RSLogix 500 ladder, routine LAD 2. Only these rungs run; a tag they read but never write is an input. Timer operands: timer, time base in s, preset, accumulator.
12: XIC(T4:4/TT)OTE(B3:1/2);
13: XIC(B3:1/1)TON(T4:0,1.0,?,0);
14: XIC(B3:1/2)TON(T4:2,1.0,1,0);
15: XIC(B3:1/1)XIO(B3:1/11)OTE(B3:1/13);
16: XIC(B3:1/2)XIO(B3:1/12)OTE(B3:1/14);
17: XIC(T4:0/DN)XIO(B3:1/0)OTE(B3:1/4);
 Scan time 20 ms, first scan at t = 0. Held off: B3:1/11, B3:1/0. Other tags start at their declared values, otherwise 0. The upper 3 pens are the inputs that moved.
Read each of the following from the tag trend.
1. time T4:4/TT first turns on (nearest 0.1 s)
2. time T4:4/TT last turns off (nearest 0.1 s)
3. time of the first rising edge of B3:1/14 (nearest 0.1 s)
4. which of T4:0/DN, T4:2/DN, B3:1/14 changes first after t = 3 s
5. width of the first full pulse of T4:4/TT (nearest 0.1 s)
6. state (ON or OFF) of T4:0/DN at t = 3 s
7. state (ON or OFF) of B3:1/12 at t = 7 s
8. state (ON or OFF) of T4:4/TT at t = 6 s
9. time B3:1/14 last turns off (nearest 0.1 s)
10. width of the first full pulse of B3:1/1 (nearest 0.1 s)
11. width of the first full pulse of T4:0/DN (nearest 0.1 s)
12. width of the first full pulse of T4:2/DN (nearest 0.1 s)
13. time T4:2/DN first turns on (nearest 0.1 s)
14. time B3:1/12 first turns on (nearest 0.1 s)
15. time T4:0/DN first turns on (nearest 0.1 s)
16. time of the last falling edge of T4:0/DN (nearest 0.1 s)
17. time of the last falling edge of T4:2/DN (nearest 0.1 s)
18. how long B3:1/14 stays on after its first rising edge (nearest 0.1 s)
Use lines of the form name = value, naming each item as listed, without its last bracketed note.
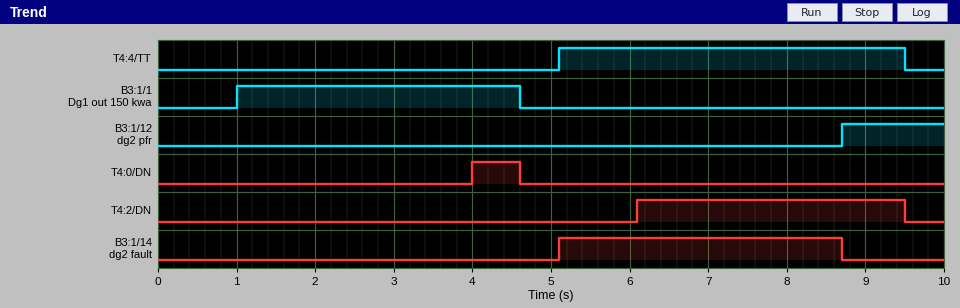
time T4:4/TT first turns on = 5.1 s
time T4:4/TT last turns off = 9.5 s
time of the first rising edge of B3:1/14 = 5.1 s
which of T4:0/DN, T4:2/DN, B3:1/14 changes first after t = 3 s = T4:0/DN
width of the first full pulse of T4:4/TT = 4.4 s
state (ON or OFF) of T4:0/DN at t = 3 s = OFF
state (ON or OFF) of B3:1/12 at t = 7 s = OFF
state (ON or OFF) of T4:4/TT at t = 6 s = ON
time B3:1/14 last turns off = 8.7 s
width of the first full pulse of B3:1/1 = 3.6 s
width of the first full pulse of T4:0/DN = 0.6 s
width of the first full pulse of T4:2/DN = 3.4 s
time T4:2/DN first turns on = 6.1 s
time B3:1/12 first turns on = 8.7 s
time T4:0/DN first turns on = 4.0 s
time of the last falling edge of T4:0/DN = 4.6 s
time of the last falling edge of T4:2/DN = 9.5 s
how long B3:1/14 stays on after its first rising edge = 3.6 s
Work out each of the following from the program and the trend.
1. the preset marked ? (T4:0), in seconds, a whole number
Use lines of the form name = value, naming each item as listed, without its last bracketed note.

the preset marked ? (T4:0), in seconds, a whole number = 3 s
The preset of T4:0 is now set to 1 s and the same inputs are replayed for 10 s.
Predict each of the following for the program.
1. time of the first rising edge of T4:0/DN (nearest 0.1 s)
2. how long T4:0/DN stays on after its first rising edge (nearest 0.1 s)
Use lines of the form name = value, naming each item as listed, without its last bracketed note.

time of the first rising edge of T4:0/DN = 2.0 s
how long T4:0/DN stays on after its first rising edge = 2.6 s
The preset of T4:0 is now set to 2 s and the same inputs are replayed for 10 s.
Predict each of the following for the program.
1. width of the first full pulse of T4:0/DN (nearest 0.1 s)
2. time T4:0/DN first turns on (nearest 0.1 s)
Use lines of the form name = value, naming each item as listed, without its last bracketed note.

width of the first full pulse of T4:0/DN = 1.6 s
time T4:0/DN first turns on = 3.0 s
